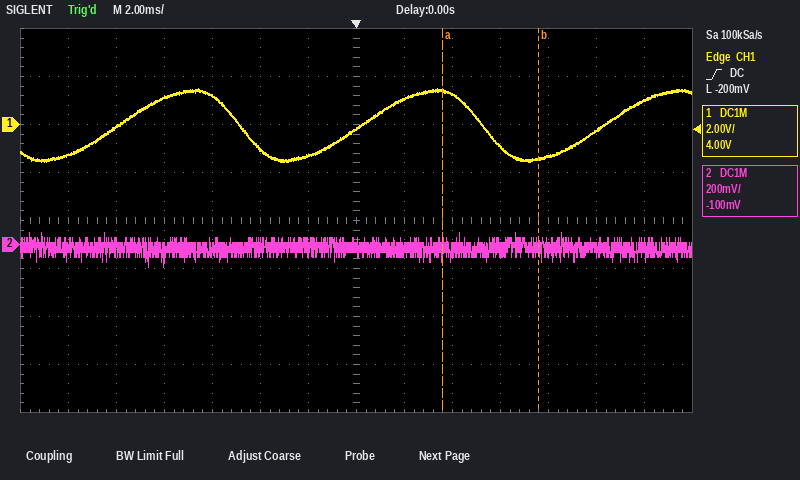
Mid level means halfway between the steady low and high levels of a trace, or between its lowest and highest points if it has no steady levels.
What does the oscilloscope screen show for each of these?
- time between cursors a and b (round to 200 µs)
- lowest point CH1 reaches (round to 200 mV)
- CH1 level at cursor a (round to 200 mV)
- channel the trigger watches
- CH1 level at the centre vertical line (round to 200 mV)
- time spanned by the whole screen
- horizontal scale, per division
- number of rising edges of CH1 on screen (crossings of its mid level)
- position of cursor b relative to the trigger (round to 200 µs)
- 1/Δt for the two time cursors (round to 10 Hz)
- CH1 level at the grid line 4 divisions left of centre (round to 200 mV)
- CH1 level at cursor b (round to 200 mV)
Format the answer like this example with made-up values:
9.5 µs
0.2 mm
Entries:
4.0 ms
-1.6 V
1.4 V
CH1
-200 mV
28 ms
2 ms
3
+7.6 ms
250 Hz
1.2 V
-1.4 V
